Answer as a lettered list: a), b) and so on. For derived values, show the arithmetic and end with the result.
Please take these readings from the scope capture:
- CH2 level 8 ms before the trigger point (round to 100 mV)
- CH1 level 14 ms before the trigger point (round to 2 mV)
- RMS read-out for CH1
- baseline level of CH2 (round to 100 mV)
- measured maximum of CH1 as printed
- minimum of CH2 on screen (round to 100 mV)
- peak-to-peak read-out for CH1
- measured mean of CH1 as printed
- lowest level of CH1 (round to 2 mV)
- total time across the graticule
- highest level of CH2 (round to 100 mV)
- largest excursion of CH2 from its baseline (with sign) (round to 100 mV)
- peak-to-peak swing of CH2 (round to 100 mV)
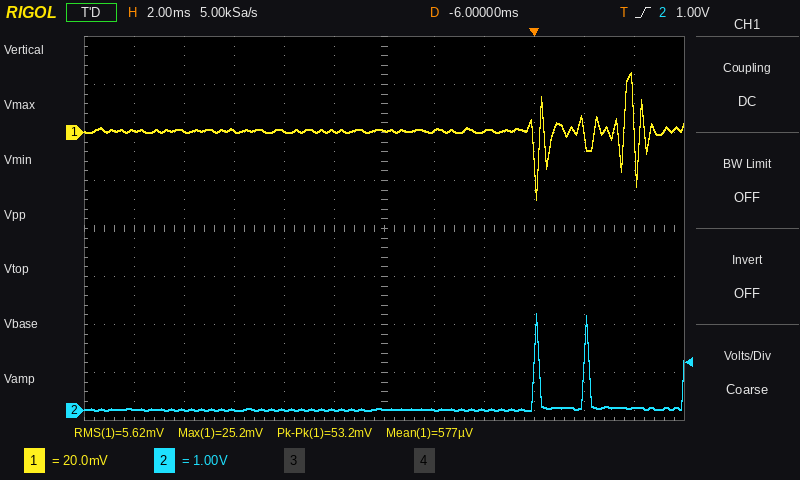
a) 0.0 V
b) 0 mV
c) 5.62 mV
d) 0.0 V
e) 25.2 mV
f) 0.0 V
g) 53.2 mV
h) 577 µV
i) -28 mV
j) 24 ms
k) 2.0 V
l) 2.0 V − (0.0 V) = +2.0 V
m) 2.0 V − (0.0 V) = 2.0 V
